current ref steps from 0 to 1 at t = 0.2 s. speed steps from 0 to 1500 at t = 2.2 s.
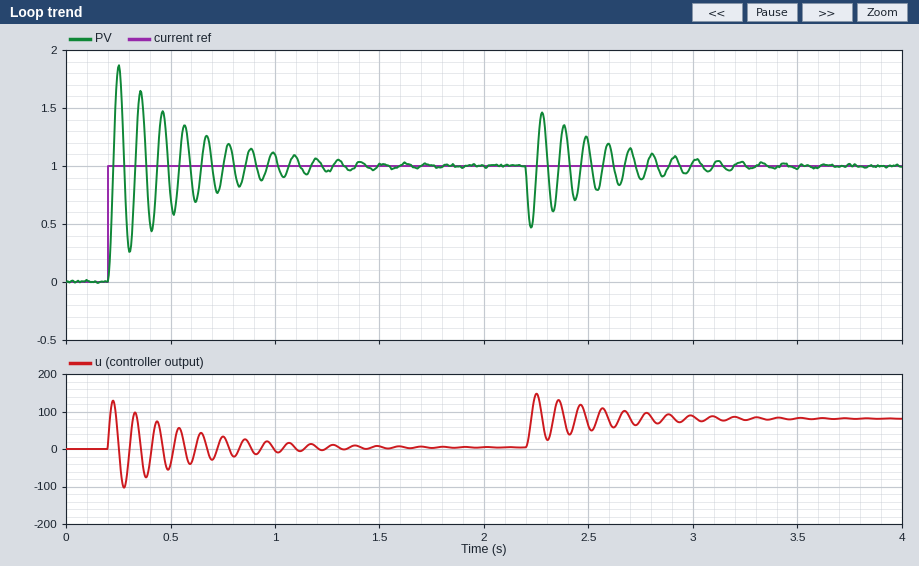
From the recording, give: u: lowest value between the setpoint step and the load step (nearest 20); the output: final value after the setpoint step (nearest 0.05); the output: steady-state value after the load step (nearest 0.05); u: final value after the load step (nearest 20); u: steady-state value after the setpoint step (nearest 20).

-100
1.00
1.00
80
0
